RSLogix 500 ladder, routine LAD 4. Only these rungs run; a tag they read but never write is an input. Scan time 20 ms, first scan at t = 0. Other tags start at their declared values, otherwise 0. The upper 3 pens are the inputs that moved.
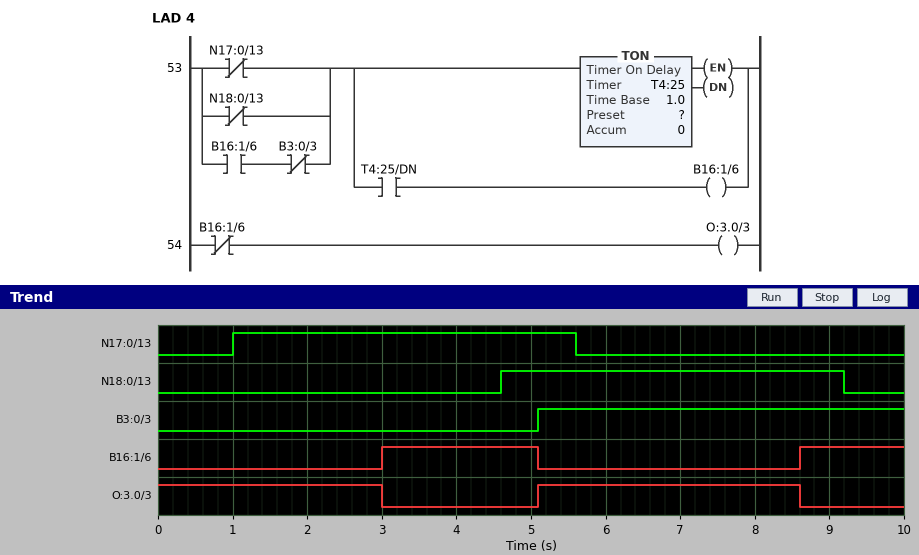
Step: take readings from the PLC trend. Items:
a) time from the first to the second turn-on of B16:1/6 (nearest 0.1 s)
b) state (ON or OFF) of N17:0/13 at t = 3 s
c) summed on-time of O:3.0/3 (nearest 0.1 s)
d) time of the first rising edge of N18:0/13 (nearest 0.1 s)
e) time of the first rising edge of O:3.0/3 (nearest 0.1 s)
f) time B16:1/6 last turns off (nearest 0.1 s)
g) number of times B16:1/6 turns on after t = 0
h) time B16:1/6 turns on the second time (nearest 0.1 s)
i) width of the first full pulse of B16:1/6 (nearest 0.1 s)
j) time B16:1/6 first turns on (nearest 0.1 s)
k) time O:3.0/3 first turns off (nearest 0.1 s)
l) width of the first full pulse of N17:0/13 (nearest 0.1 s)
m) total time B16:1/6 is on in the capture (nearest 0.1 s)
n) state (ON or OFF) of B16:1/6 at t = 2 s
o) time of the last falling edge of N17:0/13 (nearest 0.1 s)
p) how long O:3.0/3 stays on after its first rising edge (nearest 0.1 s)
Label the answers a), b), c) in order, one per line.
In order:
a) 5.6 s
b) ON
c) 6.5 s
d) 4.6 s
e) 5.1 s
f) 5.1 s
g) 2
h) 8.6 s
i) 2.1 s
j) 3.0 s
k) 3.0 s
l) 4.6 s
m) 3.5 s
n) OFF
o) 5.6 s
p) 3.5 s
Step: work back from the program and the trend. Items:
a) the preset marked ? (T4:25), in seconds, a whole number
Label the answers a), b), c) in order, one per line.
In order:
a) 3 s
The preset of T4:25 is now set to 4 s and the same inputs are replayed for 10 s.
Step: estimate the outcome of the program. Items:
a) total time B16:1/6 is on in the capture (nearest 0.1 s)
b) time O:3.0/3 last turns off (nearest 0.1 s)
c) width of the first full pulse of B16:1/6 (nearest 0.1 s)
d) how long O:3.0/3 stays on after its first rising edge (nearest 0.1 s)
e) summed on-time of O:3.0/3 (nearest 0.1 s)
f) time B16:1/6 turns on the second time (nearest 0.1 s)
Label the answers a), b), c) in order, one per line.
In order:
a) 1.5 s
b) 9.6 s
c) 1.1 s
d) 4.5 s
e) 8.5 s
f) 9.6 s
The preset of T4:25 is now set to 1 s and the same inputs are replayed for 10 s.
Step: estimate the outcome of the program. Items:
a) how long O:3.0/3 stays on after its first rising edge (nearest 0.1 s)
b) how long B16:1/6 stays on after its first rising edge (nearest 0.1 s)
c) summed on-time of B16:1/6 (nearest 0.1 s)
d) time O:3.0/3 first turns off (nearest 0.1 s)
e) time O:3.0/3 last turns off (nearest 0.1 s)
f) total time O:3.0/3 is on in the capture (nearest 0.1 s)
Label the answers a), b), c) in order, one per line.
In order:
a) 1.5 s
b) 4.1 s
c) 7.5 s
d) 1.0 s
e) 6.6 s
f) 2.5 s
